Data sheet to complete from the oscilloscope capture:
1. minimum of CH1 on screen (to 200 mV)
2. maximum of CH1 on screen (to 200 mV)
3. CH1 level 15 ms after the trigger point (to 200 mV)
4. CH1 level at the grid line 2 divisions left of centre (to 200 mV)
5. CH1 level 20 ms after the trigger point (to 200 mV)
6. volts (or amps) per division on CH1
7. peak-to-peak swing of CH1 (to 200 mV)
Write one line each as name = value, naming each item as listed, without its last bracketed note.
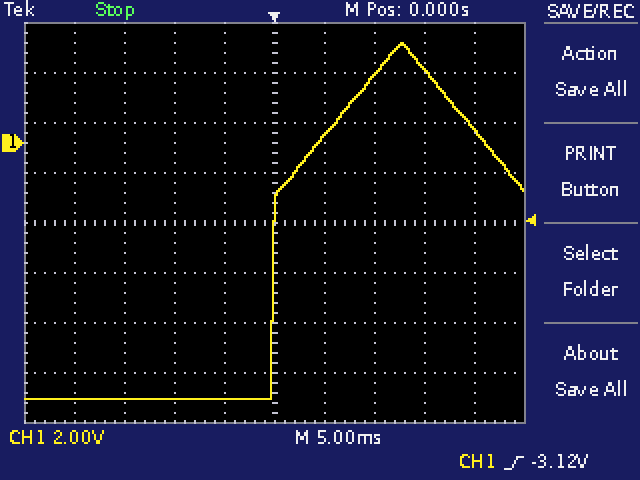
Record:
minimum of CH1 on screen = -10.2 V
maximum of CH1 on screen = 4.0 V
CH1 level 15 ms after the trigger point = 3.0 V
CH1 level at the grid line 2 divisions left of centre = -10.2 V
CH1 level 20 ms after the trigger point = 600 mV
volts (or amps) per division on CH1 = 2 V
peak-to-peak swing of CH1 = 14.2 V
